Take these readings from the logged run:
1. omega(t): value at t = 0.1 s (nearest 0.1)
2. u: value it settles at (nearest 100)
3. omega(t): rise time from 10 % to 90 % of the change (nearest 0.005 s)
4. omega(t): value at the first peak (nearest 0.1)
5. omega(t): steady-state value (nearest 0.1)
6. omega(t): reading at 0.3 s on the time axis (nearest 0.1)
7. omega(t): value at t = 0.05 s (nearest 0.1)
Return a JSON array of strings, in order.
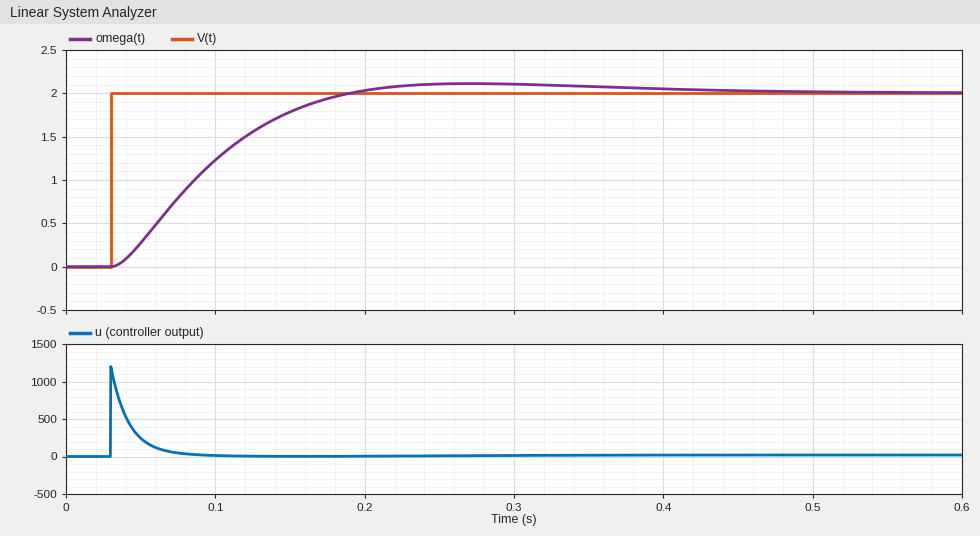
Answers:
["1.2", "0", "0.105 s", "2.1", "2.0", "2.1", "0.3"]
